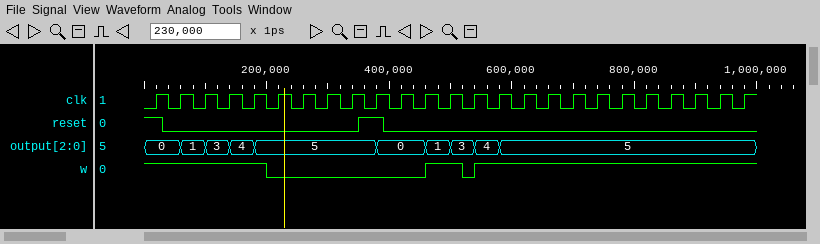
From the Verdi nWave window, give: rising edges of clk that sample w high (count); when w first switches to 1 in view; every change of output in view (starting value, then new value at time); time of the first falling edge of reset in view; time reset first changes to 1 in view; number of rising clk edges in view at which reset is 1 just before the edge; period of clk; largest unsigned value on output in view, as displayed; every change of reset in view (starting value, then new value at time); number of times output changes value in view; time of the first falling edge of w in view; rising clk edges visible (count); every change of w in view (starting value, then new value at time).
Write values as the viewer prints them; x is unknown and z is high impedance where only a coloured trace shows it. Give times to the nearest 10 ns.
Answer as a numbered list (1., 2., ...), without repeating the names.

1. 17
2. 460 ns
3. 0, 1 at 60 ns, 3 at 100 ns, 4 at 140 ns, 5 at 180 ns, 0 at 380 ns, 1 at 460 ns, 3 at 500 ns, 4 at 540 ns, 5 at 580 ns
4. 30 ns
5. 350 ns
6. 2
7. 40 ns
8. 5
9. 1, 0 at 30 ns, 1 at 350 ns, 0 at 390 ns
10. 9
11. 200 ns
12. 25
13. 1, 0 at 200 ns, 1 at 460 ns, 0 at 520 ns, 1 at 540 ns
